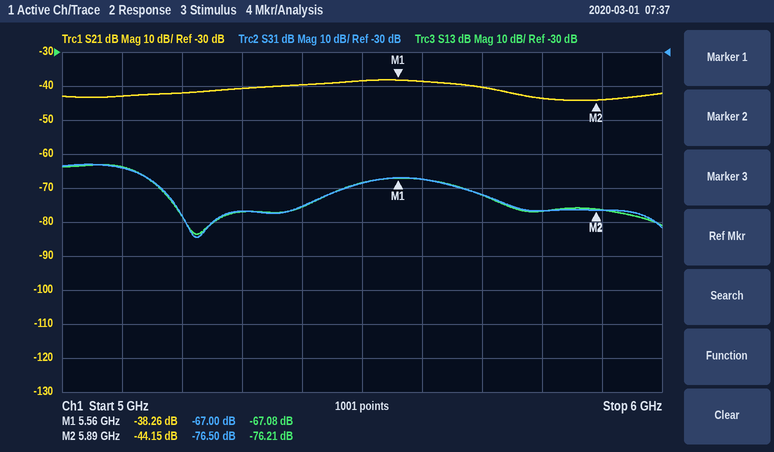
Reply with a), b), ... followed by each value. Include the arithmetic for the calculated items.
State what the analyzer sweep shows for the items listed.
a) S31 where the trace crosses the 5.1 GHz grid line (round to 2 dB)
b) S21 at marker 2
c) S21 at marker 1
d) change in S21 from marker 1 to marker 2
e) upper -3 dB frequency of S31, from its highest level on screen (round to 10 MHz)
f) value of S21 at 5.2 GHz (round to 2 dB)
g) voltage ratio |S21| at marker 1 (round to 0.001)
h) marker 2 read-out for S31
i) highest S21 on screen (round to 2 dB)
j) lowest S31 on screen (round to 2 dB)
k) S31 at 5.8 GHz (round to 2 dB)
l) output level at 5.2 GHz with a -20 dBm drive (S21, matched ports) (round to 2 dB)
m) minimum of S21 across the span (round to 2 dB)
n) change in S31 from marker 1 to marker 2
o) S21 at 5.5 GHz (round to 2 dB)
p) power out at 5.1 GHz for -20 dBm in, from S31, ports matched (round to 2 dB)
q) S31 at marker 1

a) -64 dB
b) -44.15 dB
c) -38.26 dB
d) -44.15 − (-38.26) = -5.89 dB
e) 5.13 GHz
f) -42 dB
g) 10^(-38.26/20) ≈ 0.012
h) -76.50 dB
i) -38 dB
j) -84 dB
k) -76 dB
l) -20 dBm + (-42 dB) = -62 dBm
m) -44 dB
n) -76.5 − (-67) = -9.50 dB
o) -38 dB
p) -20 dBm + (-64 dB) = -84 dBm
q) -67.00 dB
